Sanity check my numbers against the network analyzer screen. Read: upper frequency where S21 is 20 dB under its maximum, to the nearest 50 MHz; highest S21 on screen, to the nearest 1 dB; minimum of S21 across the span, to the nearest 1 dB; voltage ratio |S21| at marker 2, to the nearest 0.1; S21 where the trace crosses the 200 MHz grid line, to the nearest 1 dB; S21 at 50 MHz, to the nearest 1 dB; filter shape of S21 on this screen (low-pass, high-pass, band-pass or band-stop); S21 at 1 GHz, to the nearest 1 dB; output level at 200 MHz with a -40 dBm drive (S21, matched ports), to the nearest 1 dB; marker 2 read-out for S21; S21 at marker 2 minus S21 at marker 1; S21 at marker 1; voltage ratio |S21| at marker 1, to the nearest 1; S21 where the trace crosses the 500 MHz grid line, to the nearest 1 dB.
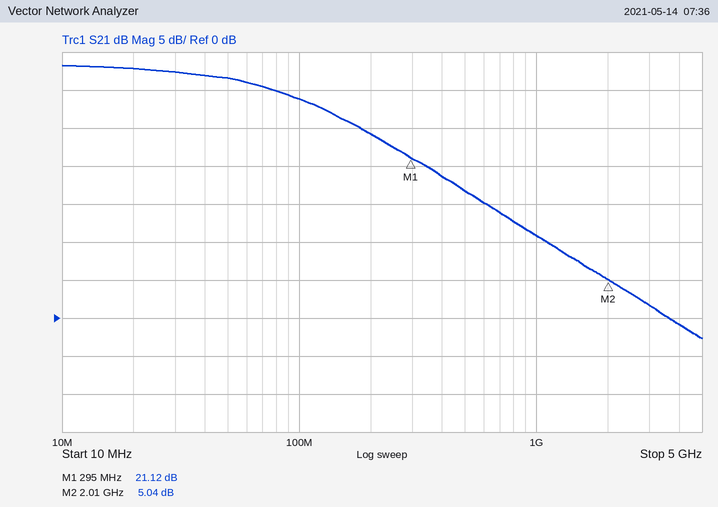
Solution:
750 MHz
33 dB
-3 dB
1.8
24 dB
32 dB
low-pass
11 dB
-16 dBm
5.04 dB
-16.08 dB
21.12 dB
11
17 dB
